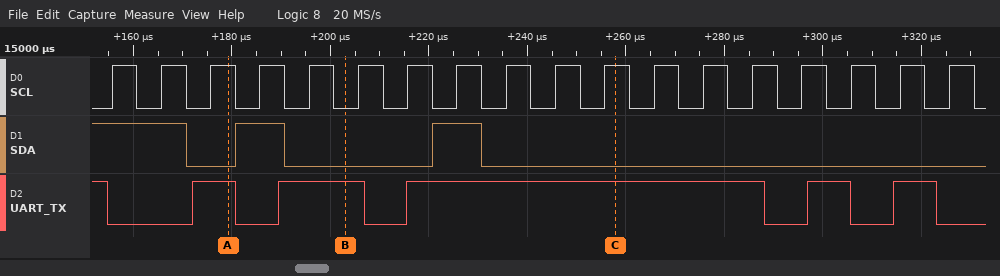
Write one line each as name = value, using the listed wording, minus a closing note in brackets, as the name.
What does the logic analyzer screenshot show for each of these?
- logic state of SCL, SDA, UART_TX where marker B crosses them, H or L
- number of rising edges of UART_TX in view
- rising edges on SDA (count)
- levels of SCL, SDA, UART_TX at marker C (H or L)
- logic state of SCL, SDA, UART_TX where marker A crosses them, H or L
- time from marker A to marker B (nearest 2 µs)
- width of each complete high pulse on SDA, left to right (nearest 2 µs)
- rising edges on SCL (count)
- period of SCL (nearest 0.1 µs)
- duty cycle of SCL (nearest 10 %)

logic state of SCL, SDA, UART_TX where marker B crosses them, H or L = SCL=L, SDA=L, UART_TX=H
number of rising edges of UART_TX in view = 5
rising edges on SDA = 2
levels of SCL, SDA, UART_TX at marker C = SCL=H, SDA=L, UART_TX=H
logic state of SCL, SDA, UART_TX where marker A crosses them, H or L = SCL=H, SDA=L, UART_TX=H
time from marker A to marker B = 24 µs
width of each complete high pulse on SDA, left to right = 10 µs, 10 µs
rising edges on SCL = 18
period of SCL = 10 µs
duty cycle of SCL = 50 %
